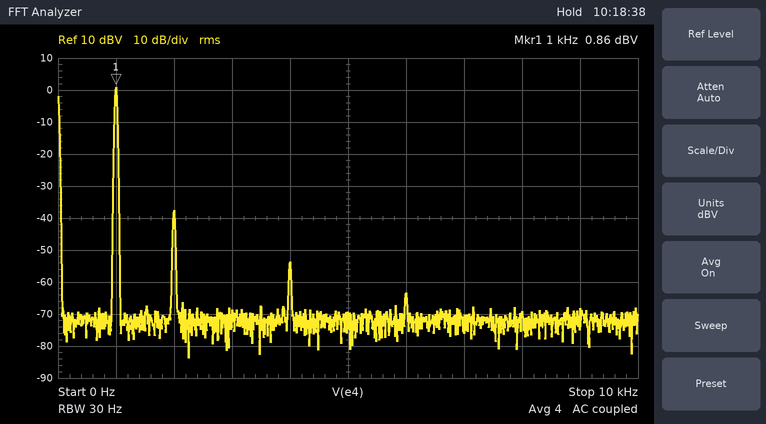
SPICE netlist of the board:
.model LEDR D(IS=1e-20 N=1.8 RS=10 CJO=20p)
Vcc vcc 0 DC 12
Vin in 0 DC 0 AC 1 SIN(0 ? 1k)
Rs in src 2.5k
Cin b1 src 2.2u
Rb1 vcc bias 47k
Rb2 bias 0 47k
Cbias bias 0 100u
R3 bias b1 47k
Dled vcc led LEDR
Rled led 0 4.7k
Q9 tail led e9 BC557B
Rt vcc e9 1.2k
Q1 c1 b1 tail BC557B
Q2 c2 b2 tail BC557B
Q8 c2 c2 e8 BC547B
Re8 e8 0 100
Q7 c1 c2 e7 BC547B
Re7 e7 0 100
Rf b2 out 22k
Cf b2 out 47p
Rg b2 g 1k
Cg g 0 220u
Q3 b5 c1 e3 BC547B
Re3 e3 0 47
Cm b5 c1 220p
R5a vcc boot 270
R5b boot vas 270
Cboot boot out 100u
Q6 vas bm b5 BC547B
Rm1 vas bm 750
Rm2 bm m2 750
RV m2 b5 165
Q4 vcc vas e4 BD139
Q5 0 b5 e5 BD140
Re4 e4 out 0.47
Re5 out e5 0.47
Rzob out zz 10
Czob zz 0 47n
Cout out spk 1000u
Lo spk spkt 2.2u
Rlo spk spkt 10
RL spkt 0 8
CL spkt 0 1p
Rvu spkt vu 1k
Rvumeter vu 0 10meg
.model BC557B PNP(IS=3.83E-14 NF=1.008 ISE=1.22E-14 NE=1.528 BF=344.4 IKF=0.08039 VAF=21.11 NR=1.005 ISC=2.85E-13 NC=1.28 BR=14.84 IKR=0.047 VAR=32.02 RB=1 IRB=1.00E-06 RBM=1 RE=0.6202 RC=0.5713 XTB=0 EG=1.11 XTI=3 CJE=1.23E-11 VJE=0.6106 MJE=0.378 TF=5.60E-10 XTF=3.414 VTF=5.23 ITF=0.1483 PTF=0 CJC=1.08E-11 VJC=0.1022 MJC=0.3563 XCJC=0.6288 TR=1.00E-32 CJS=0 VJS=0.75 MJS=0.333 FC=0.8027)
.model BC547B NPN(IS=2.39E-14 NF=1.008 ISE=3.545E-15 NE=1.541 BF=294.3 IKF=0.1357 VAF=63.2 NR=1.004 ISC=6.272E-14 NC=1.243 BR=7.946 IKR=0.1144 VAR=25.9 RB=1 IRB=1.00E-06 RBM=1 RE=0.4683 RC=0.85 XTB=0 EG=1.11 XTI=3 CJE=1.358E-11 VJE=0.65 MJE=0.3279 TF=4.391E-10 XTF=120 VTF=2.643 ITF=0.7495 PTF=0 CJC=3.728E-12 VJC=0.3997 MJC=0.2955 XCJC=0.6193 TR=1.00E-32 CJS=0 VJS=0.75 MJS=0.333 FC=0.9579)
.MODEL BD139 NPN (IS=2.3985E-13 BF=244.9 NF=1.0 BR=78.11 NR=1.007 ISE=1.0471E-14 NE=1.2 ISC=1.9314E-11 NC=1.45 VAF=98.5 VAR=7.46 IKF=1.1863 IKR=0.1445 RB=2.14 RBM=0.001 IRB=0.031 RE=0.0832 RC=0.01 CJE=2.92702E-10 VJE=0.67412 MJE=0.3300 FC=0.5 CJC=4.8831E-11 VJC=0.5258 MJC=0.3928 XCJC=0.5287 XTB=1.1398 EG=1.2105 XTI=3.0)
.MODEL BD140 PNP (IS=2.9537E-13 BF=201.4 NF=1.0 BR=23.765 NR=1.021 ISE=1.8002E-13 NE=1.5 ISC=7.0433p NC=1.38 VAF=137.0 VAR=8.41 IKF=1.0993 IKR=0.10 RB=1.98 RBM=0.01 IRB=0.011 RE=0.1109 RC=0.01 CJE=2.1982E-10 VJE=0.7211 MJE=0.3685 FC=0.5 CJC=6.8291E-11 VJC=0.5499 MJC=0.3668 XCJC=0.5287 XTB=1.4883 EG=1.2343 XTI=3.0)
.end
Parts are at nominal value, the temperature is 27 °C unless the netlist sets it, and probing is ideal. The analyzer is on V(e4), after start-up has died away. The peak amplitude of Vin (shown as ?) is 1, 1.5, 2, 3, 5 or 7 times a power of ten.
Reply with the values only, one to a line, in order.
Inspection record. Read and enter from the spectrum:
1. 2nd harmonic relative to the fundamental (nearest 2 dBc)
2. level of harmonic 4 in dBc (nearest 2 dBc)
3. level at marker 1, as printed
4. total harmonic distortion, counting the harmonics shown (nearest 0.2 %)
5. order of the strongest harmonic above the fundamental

-38 dBc
-54 dBc
0.86 dBV
1.2 %
2
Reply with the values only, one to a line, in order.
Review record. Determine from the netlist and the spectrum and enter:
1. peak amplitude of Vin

70 mV
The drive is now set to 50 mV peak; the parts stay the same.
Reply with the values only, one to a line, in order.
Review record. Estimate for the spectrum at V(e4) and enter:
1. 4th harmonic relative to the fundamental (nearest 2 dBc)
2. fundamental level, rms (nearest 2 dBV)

-56 dBc
-2 dBV
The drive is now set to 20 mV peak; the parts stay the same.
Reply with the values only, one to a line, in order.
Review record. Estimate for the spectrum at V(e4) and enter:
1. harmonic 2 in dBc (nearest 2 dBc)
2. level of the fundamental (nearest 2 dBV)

-42 dBc
-10 dBV
